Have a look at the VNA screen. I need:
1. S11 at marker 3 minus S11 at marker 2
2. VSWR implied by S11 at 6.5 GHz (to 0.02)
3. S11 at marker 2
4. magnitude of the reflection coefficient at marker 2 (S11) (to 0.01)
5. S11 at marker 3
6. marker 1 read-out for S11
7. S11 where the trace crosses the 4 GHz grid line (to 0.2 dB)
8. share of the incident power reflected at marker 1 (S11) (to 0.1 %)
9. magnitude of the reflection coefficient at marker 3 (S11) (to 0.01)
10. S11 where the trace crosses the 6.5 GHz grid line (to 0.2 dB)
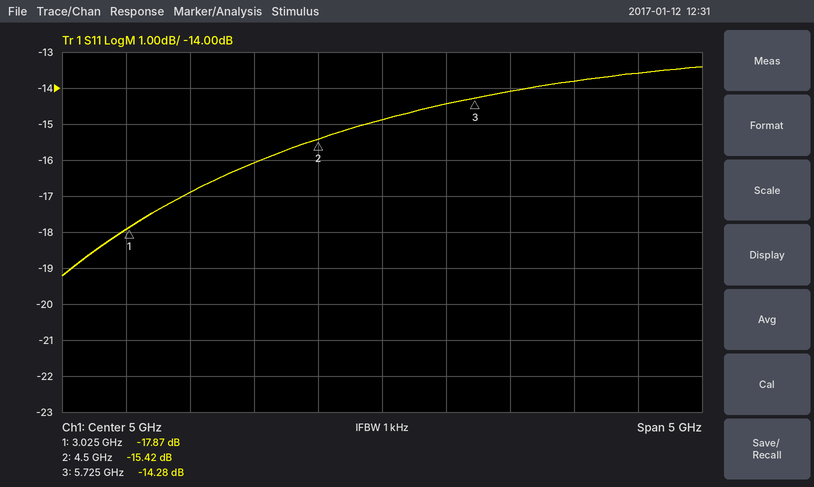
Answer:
1.14 dB
1.52
-15.42 dB
0.17
-14.28 dB
-17.87 dB
-16.0 dB
1.6 %
0.19
-13.8 dB
